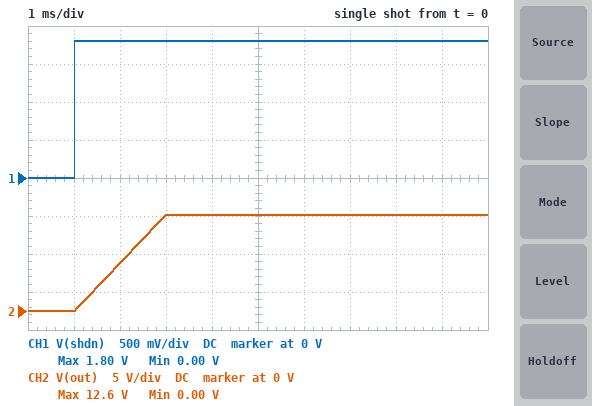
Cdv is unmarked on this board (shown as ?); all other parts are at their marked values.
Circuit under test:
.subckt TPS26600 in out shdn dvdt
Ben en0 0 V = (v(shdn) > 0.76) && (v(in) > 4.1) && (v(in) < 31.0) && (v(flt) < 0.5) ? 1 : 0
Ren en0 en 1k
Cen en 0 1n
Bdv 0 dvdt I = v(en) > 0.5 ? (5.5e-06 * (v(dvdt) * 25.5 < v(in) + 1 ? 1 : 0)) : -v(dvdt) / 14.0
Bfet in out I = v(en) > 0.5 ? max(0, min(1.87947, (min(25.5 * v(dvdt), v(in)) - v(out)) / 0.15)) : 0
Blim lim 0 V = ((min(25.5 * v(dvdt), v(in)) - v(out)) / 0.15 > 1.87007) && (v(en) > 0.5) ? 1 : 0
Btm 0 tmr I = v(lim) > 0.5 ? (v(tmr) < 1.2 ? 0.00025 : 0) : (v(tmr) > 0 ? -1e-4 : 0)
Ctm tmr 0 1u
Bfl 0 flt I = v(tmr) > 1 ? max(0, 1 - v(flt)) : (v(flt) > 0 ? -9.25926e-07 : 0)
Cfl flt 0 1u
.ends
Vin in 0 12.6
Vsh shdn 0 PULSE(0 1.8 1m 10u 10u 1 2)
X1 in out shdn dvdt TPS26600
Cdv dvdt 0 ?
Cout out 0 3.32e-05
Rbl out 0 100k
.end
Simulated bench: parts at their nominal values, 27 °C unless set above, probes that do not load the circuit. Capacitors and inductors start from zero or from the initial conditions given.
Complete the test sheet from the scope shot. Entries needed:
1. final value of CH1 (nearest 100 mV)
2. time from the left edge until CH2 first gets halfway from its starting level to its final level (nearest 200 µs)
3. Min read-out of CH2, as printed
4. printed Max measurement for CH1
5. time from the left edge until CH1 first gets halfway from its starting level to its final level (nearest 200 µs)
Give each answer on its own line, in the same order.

1.8 V
2.0 ms
0.00 V
1.80 V
1.0 ms
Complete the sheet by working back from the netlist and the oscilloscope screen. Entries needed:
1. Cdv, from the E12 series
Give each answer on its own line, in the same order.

22 nF
